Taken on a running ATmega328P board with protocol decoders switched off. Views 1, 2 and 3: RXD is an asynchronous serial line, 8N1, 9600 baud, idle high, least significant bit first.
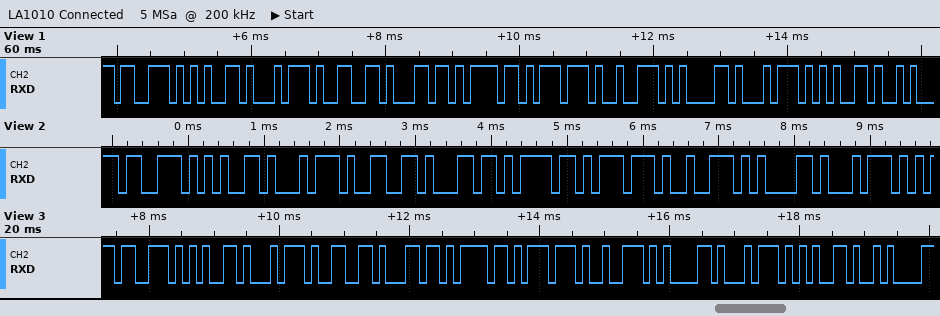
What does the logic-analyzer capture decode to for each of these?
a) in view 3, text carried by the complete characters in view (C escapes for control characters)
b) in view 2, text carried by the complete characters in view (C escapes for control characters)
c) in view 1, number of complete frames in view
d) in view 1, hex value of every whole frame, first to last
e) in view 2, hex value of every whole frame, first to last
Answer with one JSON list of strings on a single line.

["\"setflowrate\\n\"", "\"setflowrat\"", "11", "73 65 74 66 6C 6F 77 72 61 74 65", "73 65 74 66 6C 6F 77 72 61 74"]
